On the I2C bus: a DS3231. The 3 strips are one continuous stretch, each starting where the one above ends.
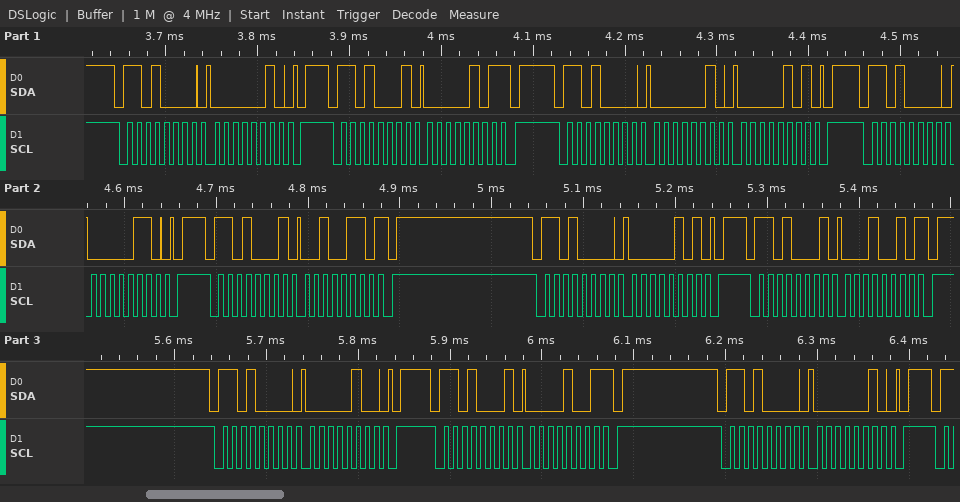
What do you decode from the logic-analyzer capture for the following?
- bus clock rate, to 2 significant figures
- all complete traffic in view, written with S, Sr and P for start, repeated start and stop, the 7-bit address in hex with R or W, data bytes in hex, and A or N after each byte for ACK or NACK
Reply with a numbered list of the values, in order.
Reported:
1. 100 kHz
2. S 68W A 02 A P S 68R A 05 N P S 68W A 02 A 05 A P S 68W A 06 A P S 68R A 26 N P S 68W A 05 A P S 68R A 12 N P S 68W A 04 A P S 68R A 09 N P S 68W A 02 A P
